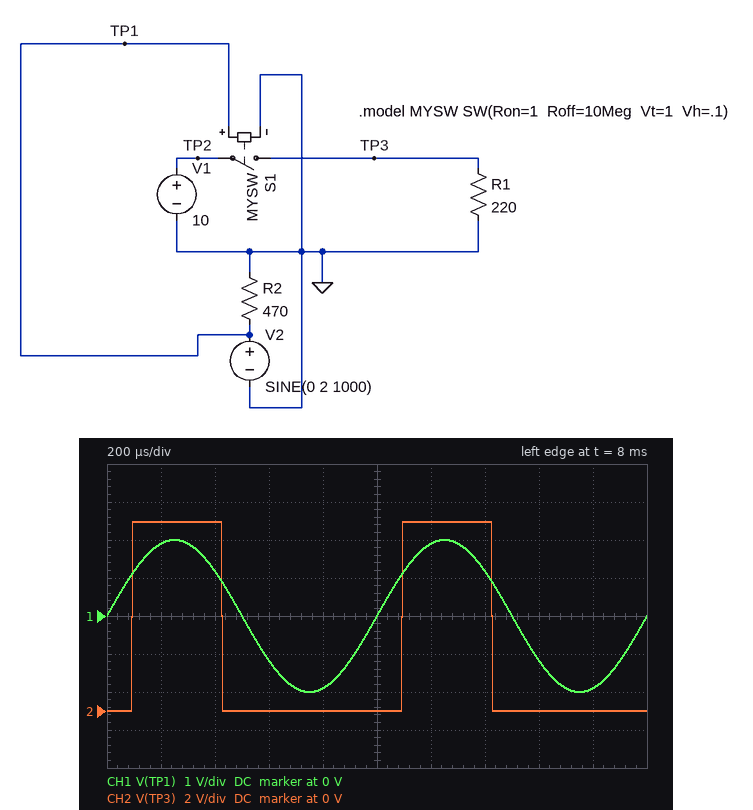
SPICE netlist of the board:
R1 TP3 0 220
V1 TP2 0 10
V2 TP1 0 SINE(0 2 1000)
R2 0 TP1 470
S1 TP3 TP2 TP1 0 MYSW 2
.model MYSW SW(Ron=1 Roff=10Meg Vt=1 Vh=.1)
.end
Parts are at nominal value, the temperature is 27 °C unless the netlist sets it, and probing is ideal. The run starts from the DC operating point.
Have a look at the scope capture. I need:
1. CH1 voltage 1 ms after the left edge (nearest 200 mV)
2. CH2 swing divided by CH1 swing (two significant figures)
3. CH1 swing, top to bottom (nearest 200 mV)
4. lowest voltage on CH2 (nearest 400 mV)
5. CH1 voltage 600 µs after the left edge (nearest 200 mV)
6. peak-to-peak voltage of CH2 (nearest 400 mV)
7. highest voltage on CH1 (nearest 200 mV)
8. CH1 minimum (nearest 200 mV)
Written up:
0 V
2.5
4.0 V
0 V
-1.2 V
10.0 V
2.0 V
-2.0 V
